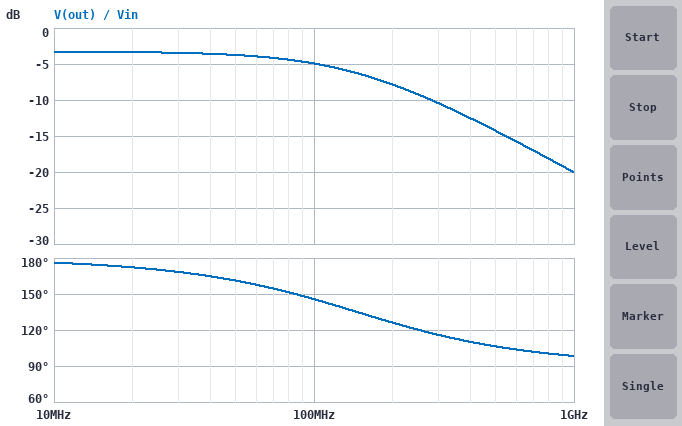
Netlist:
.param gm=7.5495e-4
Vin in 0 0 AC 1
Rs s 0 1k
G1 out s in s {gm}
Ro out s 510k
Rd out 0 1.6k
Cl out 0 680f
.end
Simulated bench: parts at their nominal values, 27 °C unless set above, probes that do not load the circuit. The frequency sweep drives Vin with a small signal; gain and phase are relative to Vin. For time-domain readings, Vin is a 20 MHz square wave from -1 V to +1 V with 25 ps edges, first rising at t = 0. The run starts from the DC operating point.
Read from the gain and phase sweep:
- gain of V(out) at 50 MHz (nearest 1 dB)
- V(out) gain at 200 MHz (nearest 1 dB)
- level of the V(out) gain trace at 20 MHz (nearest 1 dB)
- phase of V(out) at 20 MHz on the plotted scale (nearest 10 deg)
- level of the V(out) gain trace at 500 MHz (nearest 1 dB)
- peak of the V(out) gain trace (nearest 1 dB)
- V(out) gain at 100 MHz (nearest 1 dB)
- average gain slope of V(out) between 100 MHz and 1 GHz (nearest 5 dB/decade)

-4 dB
-8 dB
-3 dB
170 deg
-14 dB
-3 dB
-5 dB
-15 dB/decade
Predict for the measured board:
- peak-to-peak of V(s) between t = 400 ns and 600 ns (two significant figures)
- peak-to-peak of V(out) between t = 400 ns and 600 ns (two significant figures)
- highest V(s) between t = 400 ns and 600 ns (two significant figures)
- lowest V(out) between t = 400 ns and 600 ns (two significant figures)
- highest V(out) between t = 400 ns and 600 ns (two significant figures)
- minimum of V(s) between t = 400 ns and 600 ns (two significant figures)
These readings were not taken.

860 mV
1.4 V
430 mV
-690 mV
690 mV
-430 mV
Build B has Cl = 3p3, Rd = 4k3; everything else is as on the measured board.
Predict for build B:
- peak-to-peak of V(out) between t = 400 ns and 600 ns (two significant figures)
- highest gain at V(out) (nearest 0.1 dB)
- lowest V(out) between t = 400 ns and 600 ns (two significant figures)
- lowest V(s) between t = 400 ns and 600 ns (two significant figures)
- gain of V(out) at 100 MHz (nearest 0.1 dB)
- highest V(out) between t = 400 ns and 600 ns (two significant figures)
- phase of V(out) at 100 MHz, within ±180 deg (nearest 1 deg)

2.6 V
5.3 dB
-1.3 V
-430 mV
-13.7 dB
1.3 V
96 deg
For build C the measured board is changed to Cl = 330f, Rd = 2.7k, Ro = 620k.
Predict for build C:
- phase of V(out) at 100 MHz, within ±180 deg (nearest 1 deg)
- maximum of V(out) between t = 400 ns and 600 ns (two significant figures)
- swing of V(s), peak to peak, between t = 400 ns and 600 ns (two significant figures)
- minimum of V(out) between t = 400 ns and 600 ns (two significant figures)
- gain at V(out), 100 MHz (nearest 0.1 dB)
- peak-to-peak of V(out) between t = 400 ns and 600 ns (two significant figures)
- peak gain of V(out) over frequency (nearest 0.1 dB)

151 deg
1.2 V
860 mV
-1.2 V
0.1 dB
2.3 V
1.3 dB
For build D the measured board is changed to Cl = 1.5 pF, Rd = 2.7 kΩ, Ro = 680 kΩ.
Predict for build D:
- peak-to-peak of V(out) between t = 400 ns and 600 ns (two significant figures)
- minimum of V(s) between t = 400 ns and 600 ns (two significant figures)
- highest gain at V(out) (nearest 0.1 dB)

2.3 V
-430 mV
1.3 dB
